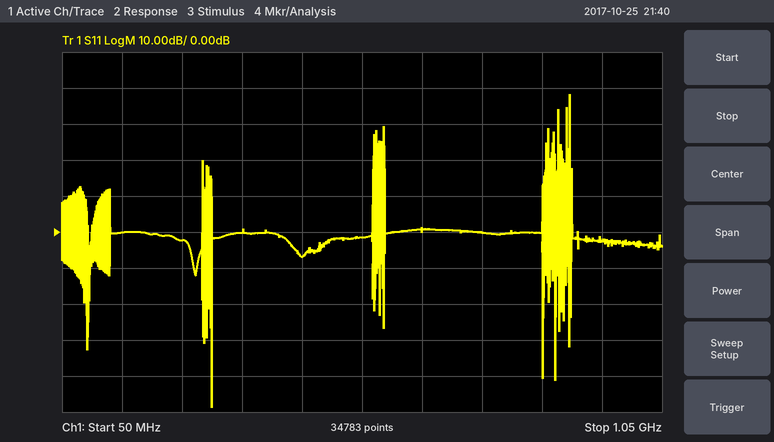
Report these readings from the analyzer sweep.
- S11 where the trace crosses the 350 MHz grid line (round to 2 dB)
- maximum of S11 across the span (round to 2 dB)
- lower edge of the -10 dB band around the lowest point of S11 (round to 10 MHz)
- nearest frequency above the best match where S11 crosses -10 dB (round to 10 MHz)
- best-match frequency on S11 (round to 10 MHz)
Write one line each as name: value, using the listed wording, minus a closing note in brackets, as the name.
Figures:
S11 where the trace crosses the 350 MHz grid line: 0 dB
maximum of S11 across the span: 38 dB
lower edge of the -10 dB band around the lowest point of S11: 300 MHz
nearest frequency above the best match where S11 crosses -10 dB: 300 MHz
best-match frequency on S11: 300 MHz
